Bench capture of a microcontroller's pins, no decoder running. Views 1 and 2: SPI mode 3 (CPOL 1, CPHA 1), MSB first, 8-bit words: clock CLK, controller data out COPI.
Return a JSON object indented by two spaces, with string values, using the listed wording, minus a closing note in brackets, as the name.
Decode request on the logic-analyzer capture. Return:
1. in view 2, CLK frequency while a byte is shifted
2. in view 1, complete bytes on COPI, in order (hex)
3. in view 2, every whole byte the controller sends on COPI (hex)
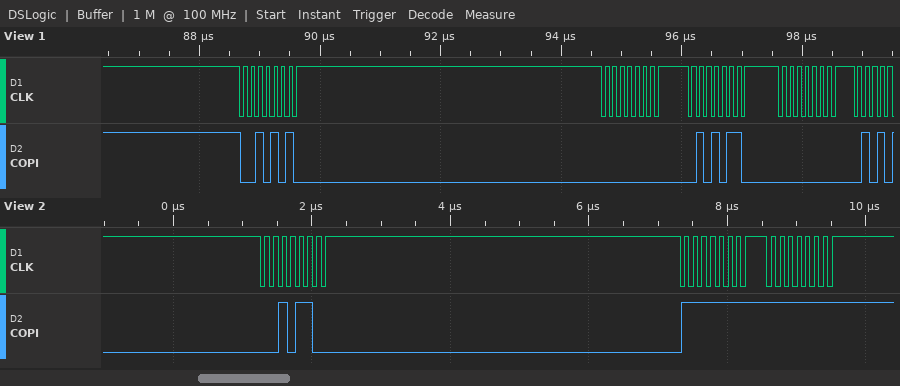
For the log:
{
  "in view 2, CLK frequency while a byte is shifted": "8 MHz",
  "in view 1, complete bytes on COPI, in order": "0x2A 0x00 0x56 0x00",
  "in view 2, every whole byte the controller sends on COPI": "2C FF FF"
}
